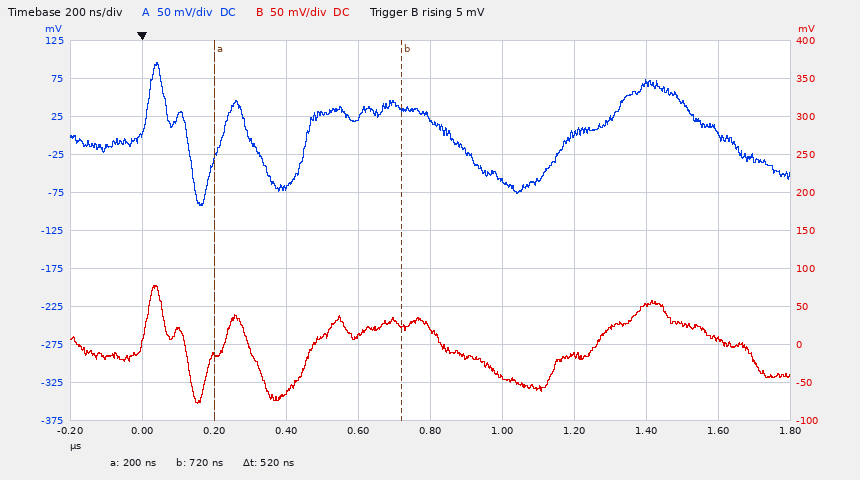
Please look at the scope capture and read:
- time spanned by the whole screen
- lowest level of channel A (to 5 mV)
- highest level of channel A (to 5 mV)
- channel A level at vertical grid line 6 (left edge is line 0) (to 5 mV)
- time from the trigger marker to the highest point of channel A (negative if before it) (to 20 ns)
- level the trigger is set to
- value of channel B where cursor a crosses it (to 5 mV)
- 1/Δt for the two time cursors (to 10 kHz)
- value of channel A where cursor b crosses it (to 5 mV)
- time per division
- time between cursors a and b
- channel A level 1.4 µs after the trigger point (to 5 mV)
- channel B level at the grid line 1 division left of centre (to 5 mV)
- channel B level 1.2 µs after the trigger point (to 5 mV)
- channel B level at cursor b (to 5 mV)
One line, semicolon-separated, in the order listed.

2 µs; -90 mV; 95 mV; -60 mV; +40 ns; 5 mV; -15 mV; 1.92 MHz; 35 mV; 200 ns; 520 ns; 70 mV; 10 mV; -15 mV; 25 mV
